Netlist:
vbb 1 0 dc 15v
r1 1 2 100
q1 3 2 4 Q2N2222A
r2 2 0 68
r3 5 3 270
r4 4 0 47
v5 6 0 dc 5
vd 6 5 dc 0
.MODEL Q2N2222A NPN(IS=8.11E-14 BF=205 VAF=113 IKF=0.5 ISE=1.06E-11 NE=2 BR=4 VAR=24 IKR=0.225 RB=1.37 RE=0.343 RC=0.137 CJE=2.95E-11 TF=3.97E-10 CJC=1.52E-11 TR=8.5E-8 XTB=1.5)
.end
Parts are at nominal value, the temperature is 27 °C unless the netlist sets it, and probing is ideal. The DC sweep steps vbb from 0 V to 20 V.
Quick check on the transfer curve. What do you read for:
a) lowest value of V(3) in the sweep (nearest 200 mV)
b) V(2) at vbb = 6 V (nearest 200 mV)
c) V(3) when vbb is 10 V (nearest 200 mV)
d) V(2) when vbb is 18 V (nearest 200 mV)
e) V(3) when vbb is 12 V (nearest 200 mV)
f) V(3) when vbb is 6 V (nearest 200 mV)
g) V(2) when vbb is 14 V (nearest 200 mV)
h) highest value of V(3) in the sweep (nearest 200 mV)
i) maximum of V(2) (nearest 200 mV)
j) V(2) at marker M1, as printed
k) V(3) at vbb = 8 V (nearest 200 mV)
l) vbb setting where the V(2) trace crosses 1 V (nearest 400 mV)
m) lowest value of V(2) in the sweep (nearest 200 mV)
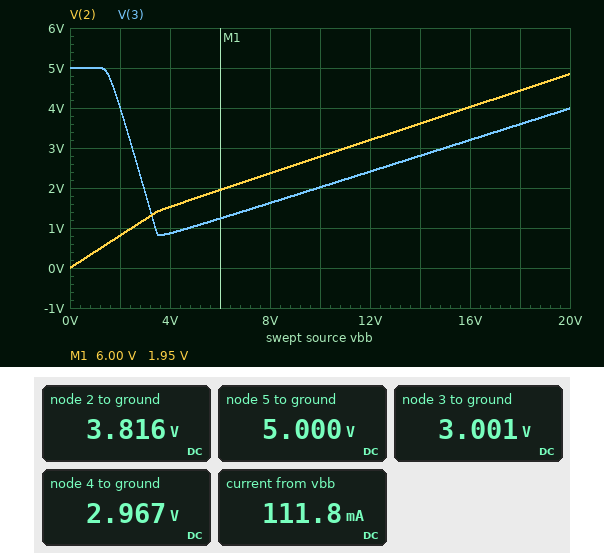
800 mV
2.0 V
2.0 V
4.4 V
2.4 V
1.2 V
3.6 V
5.0 V
4.8 V
1.95 V
1.6 V
2.4 V
0 V
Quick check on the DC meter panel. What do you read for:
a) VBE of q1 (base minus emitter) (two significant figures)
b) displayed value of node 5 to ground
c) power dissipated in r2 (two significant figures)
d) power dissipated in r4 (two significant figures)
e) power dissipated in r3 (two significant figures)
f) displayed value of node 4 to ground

850 mV
5.000 V
210 mW
190 mW
15 mW
2.967 V
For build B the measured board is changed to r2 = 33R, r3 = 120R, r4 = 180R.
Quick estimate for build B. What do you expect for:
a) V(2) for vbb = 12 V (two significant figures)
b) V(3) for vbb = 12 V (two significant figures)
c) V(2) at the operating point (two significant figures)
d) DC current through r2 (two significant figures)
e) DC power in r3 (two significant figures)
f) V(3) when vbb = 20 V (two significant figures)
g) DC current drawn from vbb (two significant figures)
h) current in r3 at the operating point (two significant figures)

3.0 V
3.5 V
3.7 V
110 mA
31 mW
3.9 V
110 mA
16 mA
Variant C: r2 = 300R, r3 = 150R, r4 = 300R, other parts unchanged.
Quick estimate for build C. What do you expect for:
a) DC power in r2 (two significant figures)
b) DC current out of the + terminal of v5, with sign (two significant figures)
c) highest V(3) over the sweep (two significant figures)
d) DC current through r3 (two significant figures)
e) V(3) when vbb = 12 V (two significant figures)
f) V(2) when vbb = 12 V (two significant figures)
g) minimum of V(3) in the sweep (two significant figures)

220 mW
-16 mA
9.5 V
16 mA
6.1 V
6.9 V
3.4 V
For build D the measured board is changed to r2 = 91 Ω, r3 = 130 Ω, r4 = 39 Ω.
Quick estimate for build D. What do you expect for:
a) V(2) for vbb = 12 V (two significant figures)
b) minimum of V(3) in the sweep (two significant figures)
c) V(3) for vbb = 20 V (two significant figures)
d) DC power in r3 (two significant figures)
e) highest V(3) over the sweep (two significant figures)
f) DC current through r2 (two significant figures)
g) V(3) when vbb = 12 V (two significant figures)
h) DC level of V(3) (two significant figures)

3.4 V
1.2 V
4.1 V
26 mW
5.0 V
44 mA
2.6 V
3.2 V
